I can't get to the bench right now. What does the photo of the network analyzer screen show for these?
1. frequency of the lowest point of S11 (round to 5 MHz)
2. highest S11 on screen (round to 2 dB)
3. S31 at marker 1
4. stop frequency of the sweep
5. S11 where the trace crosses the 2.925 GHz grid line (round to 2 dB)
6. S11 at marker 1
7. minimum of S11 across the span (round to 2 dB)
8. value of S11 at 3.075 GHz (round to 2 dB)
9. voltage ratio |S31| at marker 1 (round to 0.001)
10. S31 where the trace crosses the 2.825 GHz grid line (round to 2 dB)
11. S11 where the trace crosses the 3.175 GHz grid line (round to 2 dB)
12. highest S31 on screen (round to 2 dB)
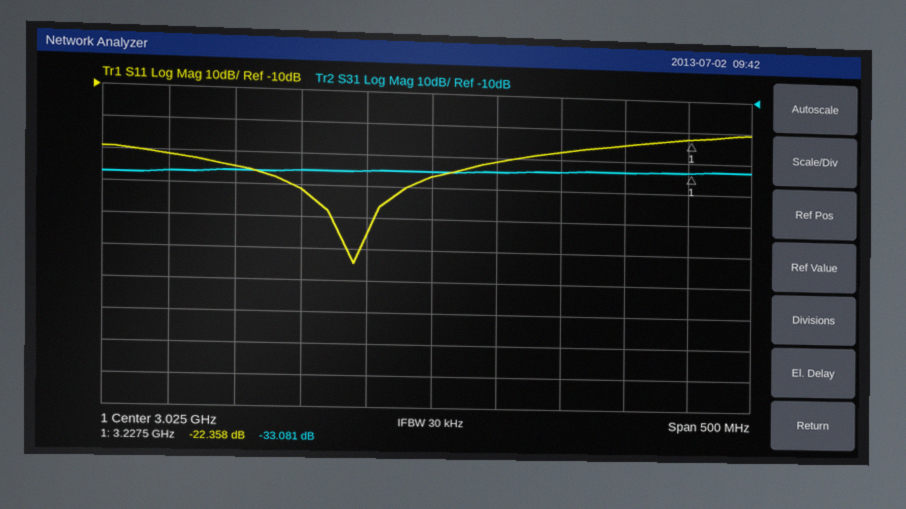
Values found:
2.965 GHz
-20 dB
-33.081 dB
3.275 GHz
-42 dB
-22.358 dB
-64 dB
-32 dB
0.022
-36 dB
-24 dB
-32 dB
